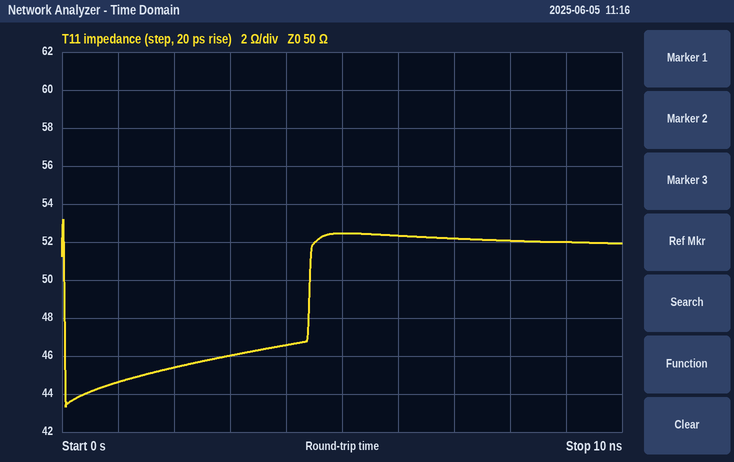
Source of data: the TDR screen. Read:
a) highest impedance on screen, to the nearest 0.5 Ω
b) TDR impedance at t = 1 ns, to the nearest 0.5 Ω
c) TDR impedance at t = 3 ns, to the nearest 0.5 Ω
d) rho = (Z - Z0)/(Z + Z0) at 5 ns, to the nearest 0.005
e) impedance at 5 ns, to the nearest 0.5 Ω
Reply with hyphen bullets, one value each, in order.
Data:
- 53.0 Ω
- 44.5 Ω
- 46.0 Ω
- +0.025
- 52.5 Ω
